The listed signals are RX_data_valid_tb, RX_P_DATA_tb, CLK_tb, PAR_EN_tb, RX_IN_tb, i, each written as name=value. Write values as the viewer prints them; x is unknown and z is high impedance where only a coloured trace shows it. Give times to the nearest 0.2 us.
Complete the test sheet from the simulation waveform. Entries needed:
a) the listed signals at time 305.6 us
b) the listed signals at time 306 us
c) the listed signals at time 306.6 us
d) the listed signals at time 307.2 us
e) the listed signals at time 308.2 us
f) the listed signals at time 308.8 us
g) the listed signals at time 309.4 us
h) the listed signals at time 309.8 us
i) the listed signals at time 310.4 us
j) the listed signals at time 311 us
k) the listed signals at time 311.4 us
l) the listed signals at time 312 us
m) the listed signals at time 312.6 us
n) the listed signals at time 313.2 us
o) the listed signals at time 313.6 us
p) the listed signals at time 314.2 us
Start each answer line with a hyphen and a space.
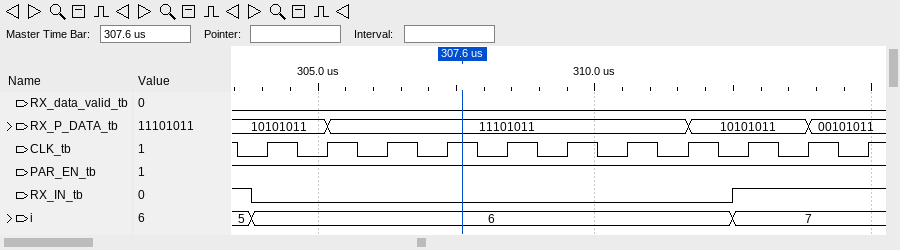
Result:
- RX_data_valid_tb=0, RX_P_DATA_tb=11101011, CLK_tb=1, PAR_EN_tb=1, RX_IN_tb=0, i=6
- RX_data_valid_tb=0, RX_P_DATA_tb=11101011, CLK_tb=0, PAR_EN_tb=1, RX_IN_tb=0, i=6
- RX_data_valid_tb=0, RX_P_DATA_tb=11101011, CLK_tb=1, PAR_EN_tb=1, RX_IN_tb=0, i=6
- RX_data_valid_tb=0, RX_P_DATA_tb=11101011, CLK_tb=0, PAR_EN_tb=1, RX_IN_tb=0, i=6
- RX_data_valid_tb=0, RX_P_DATA_tb=11101011, CLK_tb=0, PAR_EN_tb=1, RX_IN_tb=0, i=6
- RX_data_valid_tb=0, RX_P_DATA_tb=11101011, CLK_tb=1, PAR_EN_tb=1, RX_IN_tb=0, i=6
- RX_data_valid_tb=0, RX_P_DATA_tb=11101011, CLK_tb=0, PAR_EN_tb=1, RX_IN_tb=0, i=6
- RX_data_valid_tb=0, RX_P_DATA_tb=11101011, CLK_tb=1, PAR_EN_tb=1, RX_IN_tb=0, i=6
- RX_data_valid_tb=0, RX_P_DATA_tb=11101011, CLK_tb=0, PAR_EN_tb=1, RX_IN_tb=0, i=6
- RX_data_valid_tb=0, RX_P_DATA_tb=11101011, CLK_tb=1, PAR_EN_tb=1, RX_IN_tb=0, i=6
- RX_data_valid_tb=0, RX_P_DATA_tb=11101011, CLK_tb=0, PAR_EN_tb=1, RX_IN_tb=0, i=6
- RX_data_valid_tb=0, RX_P_DATA_tb=10101011, CLK_tb=1, PAR_EN_tb=1, RX_IN_tb=0, i=6
- RX_data_valid_tb=0, RX_P_DATA_tb=10101011, CLK_tb=0, PAR_EN_tb=1, RX_IN_tb=1, i=7
- RX_data_valid_tb=0, RX_P_DATA_tb=10101011, CLK_tb=1, PAR_EN_tb=1, RX_IN_tb=1, i=7
- RX_data_valid_tb=0, RX_P_DATA_tb=10101011, CLK_tb=0, PAR_EN_tb=1, RX_IN_tb=1, i=7
- RX_data_valid_tb=0, RX_P_DATA_tb=00101011, CLK_tb=1, PAR_EN_tb=1, RX_IN_tb=1, i=7
